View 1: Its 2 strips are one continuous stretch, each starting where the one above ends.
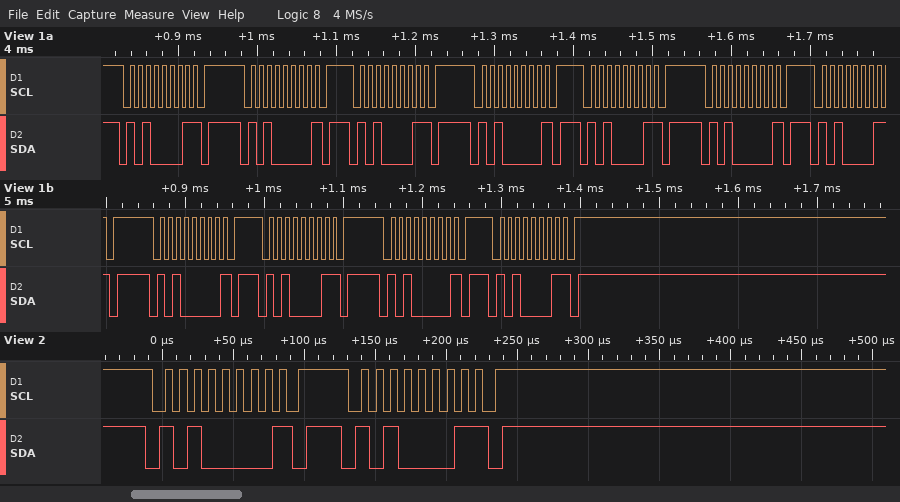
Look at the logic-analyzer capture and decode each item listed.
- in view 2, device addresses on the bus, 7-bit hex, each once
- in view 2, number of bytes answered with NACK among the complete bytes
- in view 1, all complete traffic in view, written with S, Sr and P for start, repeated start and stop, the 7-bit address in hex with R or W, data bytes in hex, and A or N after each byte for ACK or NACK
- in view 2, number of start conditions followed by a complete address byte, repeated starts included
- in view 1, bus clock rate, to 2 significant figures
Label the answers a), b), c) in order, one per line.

a) 0x50
b) 2
c) S 50R N P S 50W N P S 50R N P S 50W N P S 50R N P S 50W N P S 50R N P S 50W N P S 50R N P S 50W N P S 50R N P
d) 2
e) 100 kHz
